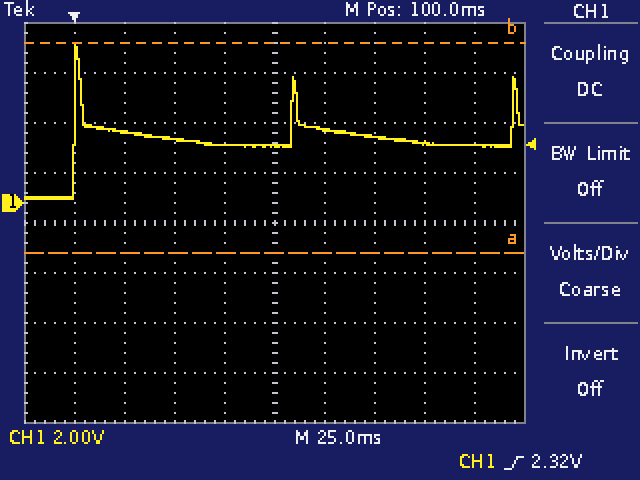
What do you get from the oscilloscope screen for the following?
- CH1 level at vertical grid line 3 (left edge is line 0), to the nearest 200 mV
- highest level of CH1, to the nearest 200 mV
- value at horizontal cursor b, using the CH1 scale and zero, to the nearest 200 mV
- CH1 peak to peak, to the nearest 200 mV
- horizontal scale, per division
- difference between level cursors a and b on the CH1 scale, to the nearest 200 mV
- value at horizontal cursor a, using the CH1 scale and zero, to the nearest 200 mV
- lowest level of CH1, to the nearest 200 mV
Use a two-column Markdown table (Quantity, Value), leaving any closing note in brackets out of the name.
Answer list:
| Quantity | Value |
|---|---|
| CH1 level at vertical grid line 3 (left edge is line 0), to the nearest 200 mV | 2.6 V |
| highest level of CH1, to the nearest 200 mV | 6.4 V |
| value at horizontal cursor b, using the CH1 scale and zero, to the nearest 200 mV | 6.4 V |
| CH1 peak to peak, to the nearest 200 mV | 6.2 V |
| horizontal scale, per division | 25 ms |
| difference between level cursors a and b on the CH1 scale, to the nearest 200 mV | 8.4 V |
| value at horizontal cursor a, using the CH1 scale and zero, to the nearest 200 mV | -2.0 V |
| lowest level of CH1, to the nearest 200 mV | 200 mV |
